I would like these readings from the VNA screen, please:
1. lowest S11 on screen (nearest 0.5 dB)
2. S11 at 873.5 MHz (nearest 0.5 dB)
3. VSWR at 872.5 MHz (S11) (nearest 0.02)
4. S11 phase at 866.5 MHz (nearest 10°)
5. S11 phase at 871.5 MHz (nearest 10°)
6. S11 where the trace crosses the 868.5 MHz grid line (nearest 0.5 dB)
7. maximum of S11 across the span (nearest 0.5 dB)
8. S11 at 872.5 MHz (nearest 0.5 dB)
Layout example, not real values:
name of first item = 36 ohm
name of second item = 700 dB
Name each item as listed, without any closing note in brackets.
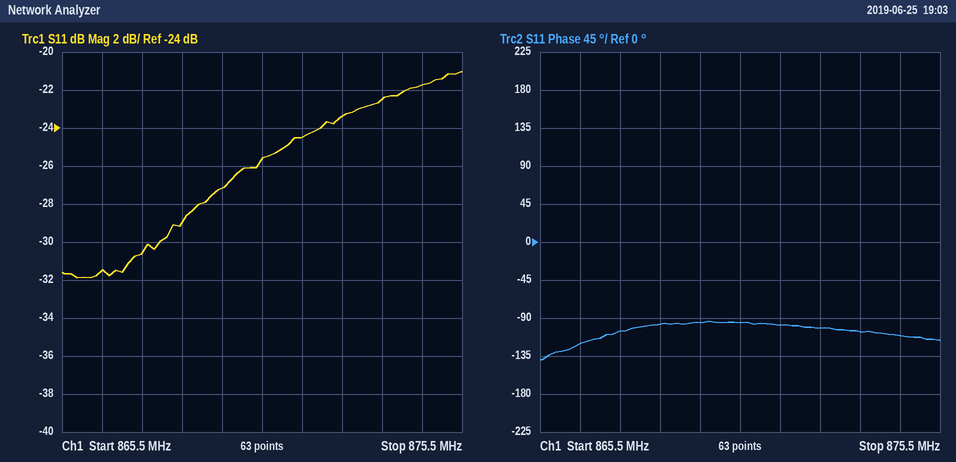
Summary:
lowest S11 on screen = -32.0 dB
S11 at 873.5 MHz = -22.5 dB
VSWR at 872.5 MHz (S11) = 1.14
S11 phase at 866.5 MHz = -120°
S11 phase at 871.5 MHz = -100°
S11 where the trace crosses the 868.5 MHz grid line = -29.0 dB
maximum of S11 across the span = -21.0 dB
S11 at 872.5 MHz = -23.5 dB
